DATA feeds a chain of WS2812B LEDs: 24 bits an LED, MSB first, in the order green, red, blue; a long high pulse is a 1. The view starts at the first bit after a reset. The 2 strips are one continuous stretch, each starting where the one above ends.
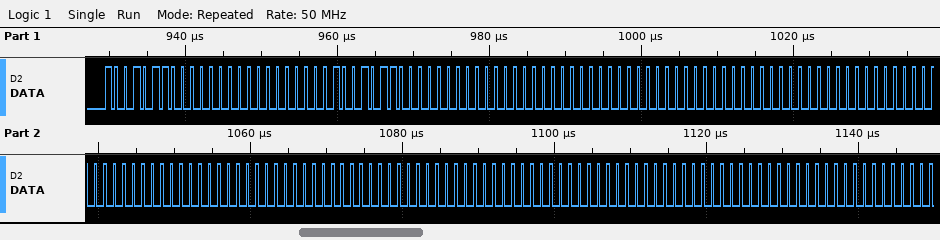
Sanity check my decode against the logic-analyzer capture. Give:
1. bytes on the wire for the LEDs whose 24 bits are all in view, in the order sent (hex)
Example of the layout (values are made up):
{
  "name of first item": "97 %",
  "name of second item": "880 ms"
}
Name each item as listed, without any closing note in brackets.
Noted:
{
  "bytes on the wire for the LEDs whose 24 bits are all in view, in the order sent": "96 00 00 96 00 00 00 00 00 00 00 00 00 00 00 00 00 00 00 00 00"
}
